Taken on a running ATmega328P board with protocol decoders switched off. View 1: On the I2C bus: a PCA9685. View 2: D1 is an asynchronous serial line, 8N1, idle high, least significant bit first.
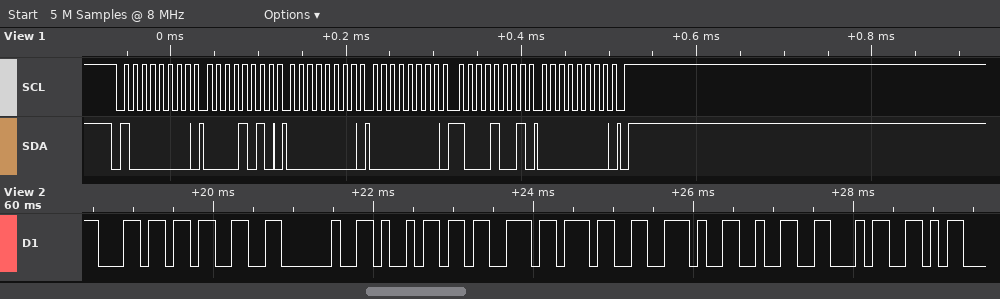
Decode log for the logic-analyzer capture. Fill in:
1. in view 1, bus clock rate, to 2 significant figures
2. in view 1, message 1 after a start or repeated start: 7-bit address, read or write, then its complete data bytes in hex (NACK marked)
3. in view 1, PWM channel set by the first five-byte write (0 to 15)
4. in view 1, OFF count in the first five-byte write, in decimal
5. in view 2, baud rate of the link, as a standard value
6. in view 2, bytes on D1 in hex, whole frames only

100 kHz
0x40 write: 0A 00 00 89 00
1
137
9600 baud
6C 33 20 69 73 37 2E 32 34
